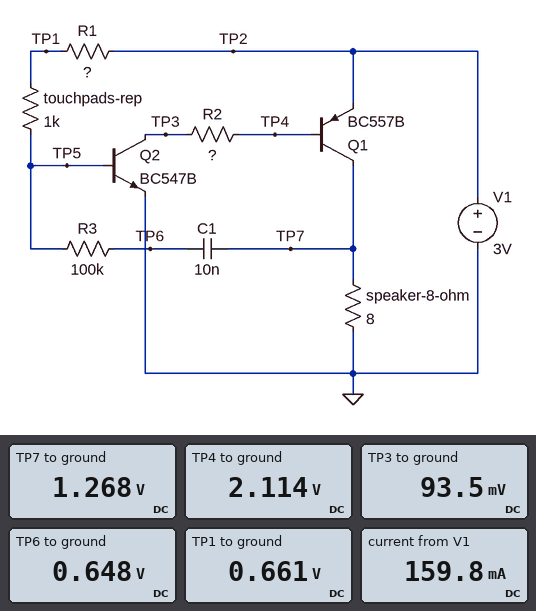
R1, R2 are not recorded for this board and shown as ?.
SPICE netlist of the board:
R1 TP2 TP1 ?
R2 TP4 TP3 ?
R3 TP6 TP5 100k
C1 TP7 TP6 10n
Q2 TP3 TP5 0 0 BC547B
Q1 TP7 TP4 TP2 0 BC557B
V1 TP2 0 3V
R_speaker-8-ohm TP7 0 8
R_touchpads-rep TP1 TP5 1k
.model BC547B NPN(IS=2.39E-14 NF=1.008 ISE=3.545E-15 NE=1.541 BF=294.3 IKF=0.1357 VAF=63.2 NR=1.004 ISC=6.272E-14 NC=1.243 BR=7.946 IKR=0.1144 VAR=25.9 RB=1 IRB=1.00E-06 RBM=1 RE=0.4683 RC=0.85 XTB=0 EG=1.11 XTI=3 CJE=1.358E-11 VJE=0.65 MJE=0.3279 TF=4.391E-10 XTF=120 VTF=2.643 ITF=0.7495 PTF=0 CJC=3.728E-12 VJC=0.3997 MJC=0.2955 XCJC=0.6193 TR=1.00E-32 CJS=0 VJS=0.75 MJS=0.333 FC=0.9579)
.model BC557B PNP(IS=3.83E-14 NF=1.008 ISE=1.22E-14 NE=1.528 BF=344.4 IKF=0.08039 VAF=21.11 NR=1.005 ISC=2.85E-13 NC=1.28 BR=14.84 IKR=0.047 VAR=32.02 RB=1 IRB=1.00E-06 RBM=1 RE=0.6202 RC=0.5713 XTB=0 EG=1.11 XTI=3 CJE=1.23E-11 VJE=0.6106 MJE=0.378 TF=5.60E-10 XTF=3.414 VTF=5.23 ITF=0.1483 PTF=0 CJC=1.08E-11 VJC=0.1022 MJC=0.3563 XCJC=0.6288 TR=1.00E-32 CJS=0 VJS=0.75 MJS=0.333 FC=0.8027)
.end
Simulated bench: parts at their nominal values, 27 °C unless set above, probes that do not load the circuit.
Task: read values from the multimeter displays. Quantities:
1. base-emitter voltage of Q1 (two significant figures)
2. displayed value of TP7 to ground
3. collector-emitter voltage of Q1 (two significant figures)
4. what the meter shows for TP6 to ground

-890 mV
1.268 V
-1.7 V
0.648 V
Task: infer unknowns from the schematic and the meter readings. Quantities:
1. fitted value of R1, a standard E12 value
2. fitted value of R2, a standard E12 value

180 kΩ
1.5 kΩ
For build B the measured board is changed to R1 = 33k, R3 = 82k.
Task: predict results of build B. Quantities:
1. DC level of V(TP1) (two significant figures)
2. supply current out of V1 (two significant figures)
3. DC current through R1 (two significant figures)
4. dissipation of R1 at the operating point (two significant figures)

720 mV
160 mA
69 µA
160 µW
